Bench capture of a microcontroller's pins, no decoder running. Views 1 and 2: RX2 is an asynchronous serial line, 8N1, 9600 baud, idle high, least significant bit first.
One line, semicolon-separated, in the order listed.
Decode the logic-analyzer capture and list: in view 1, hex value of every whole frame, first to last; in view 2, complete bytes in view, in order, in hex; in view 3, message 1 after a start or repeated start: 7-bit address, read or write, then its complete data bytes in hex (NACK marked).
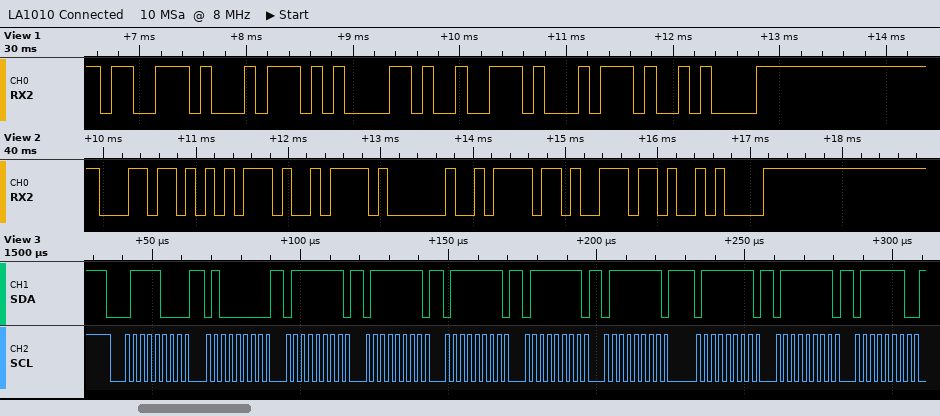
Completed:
73 74 61 72 74 0A; 0x6C 0x75 0x7A 0x20 0x6F 0x6E 0x0A; 0x3C write: 40 7F 7F 7F 7F 7F 7F 7F 7E
